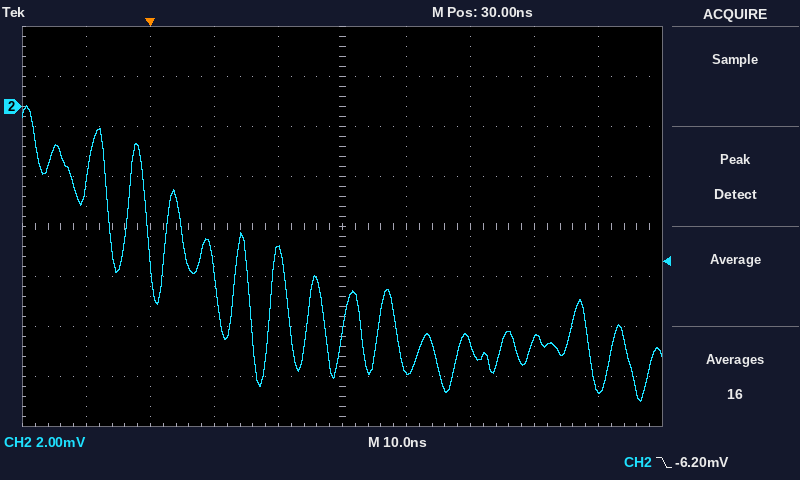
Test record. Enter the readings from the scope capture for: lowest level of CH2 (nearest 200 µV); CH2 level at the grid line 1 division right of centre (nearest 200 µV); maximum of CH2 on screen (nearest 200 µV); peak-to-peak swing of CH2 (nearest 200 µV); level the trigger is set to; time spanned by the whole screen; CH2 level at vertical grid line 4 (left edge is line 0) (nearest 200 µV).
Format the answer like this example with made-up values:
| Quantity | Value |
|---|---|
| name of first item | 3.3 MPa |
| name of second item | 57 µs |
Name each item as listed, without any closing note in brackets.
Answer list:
| Quantity | Value |
|---|---|
| lowest level of CH2 | -11.8 mV |
| CH2 level at the grid line 1 division right of centre | -10.6 mV |
| maximum of CH2 on screen | 0.0 mV |
| peak-to-peak swing of CH2 | 11.8 mV |
| level the trigger is set to | -6.20 mV |
| time spanned by the whole screen | 100 ns |
| CH2 level at vertical grid line 4 (left edge is line 0) | -5.8 mV |
